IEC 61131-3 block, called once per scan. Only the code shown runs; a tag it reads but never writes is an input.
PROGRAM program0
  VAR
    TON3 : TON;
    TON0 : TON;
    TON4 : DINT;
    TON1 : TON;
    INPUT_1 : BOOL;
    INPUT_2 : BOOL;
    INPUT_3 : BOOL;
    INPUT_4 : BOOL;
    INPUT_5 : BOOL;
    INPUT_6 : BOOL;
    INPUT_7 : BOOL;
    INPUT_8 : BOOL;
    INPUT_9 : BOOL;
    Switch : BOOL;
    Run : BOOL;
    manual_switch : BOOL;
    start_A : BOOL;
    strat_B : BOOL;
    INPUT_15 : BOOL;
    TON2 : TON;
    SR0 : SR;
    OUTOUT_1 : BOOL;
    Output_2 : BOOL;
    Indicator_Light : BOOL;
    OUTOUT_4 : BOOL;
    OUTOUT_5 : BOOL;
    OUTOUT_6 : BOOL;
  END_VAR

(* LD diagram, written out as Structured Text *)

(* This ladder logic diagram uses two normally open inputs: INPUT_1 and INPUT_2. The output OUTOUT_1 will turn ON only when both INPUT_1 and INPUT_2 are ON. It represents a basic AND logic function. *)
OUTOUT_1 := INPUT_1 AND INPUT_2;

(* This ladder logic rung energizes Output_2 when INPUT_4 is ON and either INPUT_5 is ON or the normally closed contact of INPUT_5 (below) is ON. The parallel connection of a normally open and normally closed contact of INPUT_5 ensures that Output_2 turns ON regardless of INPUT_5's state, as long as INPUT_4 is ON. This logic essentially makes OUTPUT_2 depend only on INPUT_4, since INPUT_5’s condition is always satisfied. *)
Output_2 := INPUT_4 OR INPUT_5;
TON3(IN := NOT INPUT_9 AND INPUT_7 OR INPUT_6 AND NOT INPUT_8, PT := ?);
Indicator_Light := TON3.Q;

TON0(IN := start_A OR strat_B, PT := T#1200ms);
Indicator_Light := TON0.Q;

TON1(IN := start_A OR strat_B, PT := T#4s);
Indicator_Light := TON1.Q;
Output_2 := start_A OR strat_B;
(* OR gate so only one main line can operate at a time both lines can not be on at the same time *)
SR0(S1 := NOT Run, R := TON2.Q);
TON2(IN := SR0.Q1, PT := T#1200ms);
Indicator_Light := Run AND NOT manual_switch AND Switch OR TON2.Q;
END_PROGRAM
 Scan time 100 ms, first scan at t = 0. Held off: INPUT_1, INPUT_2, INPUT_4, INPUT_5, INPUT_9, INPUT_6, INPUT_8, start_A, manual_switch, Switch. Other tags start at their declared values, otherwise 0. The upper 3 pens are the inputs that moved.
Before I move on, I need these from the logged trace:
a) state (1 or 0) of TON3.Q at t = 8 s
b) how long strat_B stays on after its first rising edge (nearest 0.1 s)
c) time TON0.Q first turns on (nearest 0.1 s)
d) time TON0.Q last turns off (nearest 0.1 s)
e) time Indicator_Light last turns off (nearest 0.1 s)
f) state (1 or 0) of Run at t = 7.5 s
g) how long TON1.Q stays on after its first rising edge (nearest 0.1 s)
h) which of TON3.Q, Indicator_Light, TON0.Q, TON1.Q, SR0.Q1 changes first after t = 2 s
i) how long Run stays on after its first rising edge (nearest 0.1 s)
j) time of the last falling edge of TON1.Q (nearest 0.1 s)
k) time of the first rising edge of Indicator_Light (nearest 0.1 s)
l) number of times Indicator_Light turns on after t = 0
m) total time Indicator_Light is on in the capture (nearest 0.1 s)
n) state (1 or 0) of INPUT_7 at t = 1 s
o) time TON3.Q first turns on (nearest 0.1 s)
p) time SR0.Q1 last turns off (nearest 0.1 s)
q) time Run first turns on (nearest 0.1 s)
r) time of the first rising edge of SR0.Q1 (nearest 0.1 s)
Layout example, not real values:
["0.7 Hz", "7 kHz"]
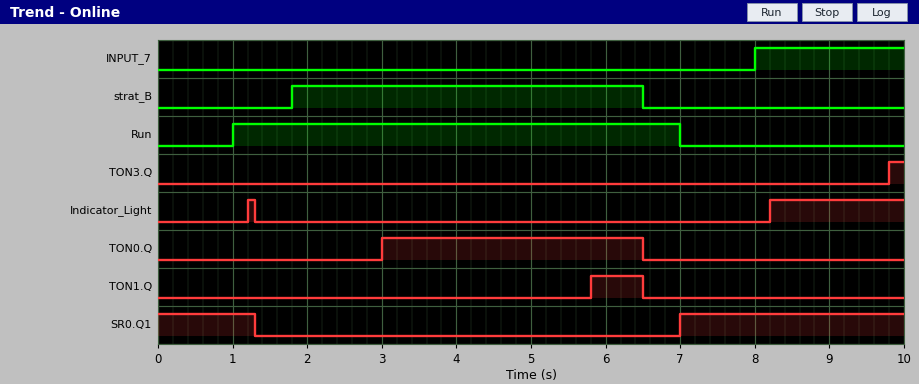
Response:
["0", "4.7 s", "3.0 s", "6.5 s", "1.3 s", "0", "0.7 s", "TON0.Q", "6.0 s", "6.5 s", "1.2 s", "2", "1.9 s", "0", "9.8 s", "1.3 s", "1.0 s", "7.0 s"]
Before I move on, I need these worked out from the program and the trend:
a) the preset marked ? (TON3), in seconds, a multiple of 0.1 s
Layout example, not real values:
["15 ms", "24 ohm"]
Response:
["1.8 s"]
